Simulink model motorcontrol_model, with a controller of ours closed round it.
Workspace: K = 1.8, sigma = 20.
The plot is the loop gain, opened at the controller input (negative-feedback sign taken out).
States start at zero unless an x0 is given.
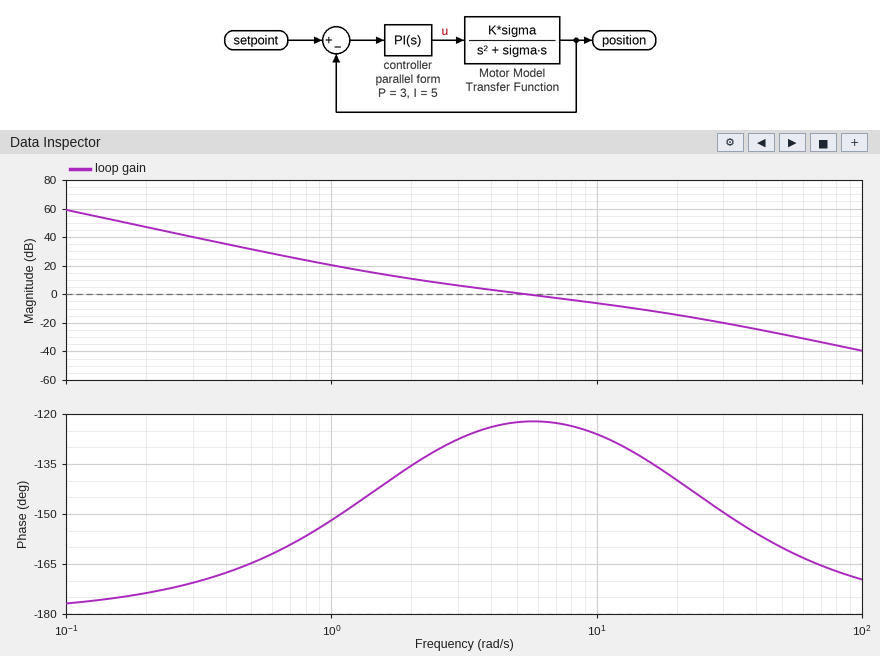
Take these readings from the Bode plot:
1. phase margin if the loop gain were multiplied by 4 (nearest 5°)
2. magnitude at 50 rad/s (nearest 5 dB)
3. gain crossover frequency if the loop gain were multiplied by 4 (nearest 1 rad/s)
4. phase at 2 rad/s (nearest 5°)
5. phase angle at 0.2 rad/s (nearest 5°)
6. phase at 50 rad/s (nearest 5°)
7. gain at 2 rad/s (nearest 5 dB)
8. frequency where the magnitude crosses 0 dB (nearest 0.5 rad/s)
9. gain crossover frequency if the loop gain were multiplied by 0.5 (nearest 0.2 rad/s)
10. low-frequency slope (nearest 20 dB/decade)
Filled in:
45°
-30 dB
17 rad/s
-135°
-175°
-160°
10 dB
5.5 rad/s
3.0 rad/s
-40 dB/decade
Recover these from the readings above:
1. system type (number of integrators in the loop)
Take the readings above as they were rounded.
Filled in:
2
